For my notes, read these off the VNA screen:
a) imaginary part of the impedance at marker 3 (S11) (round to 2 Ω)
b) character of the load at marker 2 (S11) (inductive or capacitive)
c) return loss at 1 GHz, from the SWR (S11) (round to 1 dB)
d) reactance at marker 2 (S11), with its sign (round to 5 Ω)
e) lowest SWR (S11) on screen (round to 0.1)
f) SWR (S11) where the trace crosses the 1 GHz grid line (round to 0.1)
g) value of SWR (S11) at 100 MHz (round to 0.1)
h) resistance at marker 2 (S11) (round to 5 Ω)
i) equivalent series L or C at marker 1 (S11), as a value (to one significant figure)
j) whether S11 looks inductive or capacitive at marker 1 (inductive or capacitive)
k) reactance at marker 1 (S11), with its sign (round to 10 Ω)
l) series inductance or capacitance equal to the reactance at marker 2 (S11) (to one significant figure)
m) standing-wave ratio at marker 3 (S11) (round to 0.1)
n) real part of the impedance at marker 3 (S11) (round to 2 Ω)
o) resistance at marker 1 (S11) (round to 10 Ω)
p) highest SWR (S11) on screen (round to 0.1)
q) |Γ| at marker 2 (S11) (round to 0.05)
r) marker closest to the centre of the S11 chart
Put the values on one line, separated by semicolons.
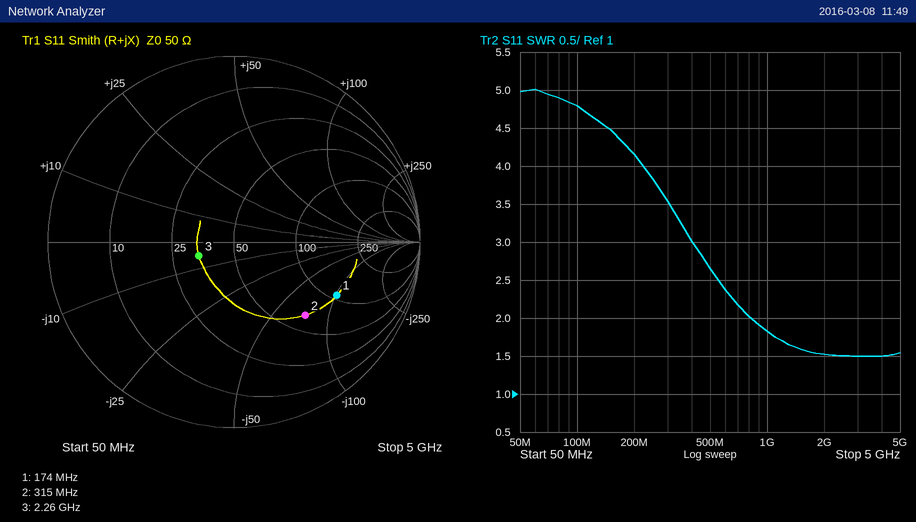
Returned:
-6 Ω; capacitive; 11 dB; -75 Ω; 1.5; 1.8; 4.8; 65 Ω; 9 pF; capacitive; -100 Ω; 7 pF; 1.5; 34 Ω; 110 Ω; 5.0; 0.55; marker 3
